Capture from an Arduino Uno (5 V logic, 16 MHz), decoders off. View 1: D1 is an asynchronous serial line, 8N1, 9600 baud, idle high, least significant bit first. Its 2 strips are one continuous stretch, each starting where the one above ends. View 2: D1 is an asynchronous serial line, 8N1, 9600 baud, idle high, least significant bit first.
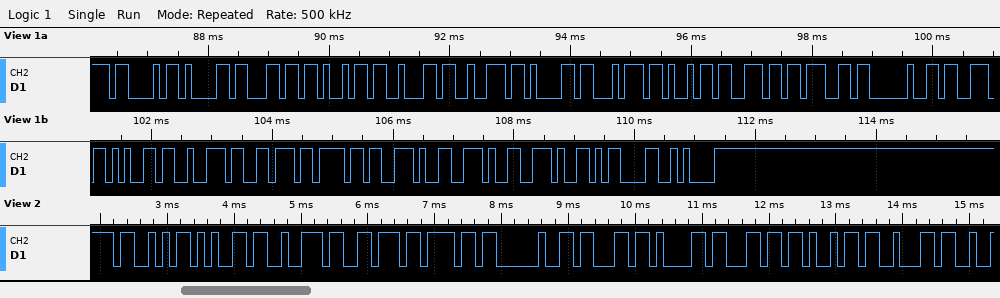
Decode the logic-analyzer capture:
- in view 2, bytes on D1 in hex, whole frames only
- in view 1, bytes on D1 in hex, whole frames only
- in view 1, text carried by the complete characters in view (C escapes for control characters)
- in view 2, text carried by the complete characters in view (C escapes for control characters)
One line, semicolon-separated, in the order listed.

0x53 0x65 0x72 0x76 0x6F 0x20 0x63 0x61 0x6C 0x69 0x62; 43 61 6C 69 62 72 61 74 69 6E 67 20 73 65 72 76 6F 2E 2E 2E 0D 0A; "Calibrating servo...\r\n"; "Servo calib"
